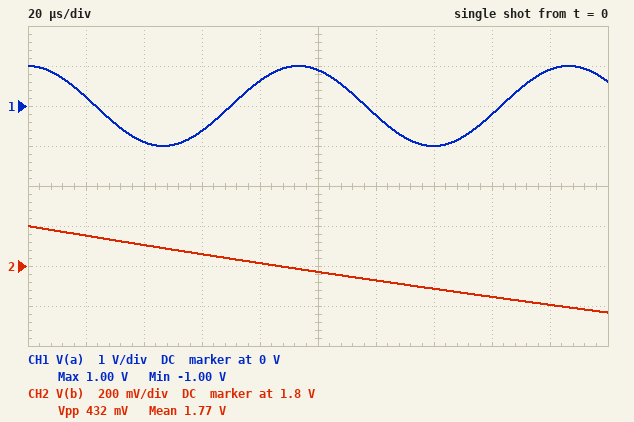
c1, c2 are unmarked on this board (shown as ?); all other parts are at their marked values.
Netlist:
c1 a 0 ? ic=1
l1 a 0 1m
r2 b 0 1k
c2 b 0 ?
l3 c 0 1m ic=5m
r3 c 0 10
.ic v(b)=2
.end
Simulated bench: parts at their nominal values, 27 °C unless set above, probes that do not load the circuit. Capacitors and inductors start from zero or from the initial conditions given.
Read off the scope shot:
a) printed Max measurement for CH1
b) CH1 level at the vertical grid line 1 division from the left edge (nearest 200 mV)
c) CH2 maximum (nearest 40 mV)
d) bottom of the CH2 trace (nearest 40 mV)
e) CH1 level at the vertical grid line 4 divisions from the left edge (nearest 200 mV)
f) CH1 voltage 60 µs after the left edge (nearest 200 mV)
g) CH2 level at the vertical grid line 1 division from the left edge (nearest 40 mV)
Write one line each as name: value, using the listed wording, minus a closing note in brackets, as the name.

printed Max measurement for CH1: 1.00 V
CH1 level at the vertical grid line 1 division from the left edge: 200 mV
CH2 maximum: 2.00 V
bottom of the CH2 trace: 1.56 V
CH1 level at the vertical grid line 4 divisions from the left edge: 600 mV
CH1 voltage 60 µs after the left edge: -600 mV
CH2 level at the vertical grid line 1 division from the left edge: 1.96 V
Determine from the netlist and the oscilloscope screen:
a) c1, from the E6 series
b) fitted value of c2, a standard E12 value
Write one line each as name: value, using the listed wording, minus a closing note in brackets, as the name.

c1, from the E6 series: 220 nF
fitted value of c2, a standard E12 value: 820 nF
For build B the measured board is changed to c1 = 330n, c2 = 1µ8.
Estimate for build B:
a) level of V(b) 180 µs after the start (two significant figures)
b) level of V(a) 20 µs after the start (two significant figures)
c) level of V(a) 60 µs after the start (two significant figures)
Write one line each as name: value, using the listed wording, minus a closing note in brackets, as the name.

level of V(b) 180 µs after the start: 1.8 V
level of V(a) 20 µs after the start: 450 mV
level of V(a) 60 µs after the start: -990 mV
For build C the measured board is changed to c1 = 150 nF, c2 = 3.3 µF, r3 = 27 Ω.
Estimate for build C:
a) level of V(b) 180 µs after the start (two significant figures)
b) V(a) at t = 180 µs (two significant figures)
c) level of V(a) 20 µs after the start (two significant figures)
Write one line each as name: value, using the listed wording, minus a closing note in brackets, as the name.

level of V(b) 180 µs after the start: 1.9 V
V(a) at t = 180 µs: -530 mV
level of V(a) 20 µs after the start: -62 mV
